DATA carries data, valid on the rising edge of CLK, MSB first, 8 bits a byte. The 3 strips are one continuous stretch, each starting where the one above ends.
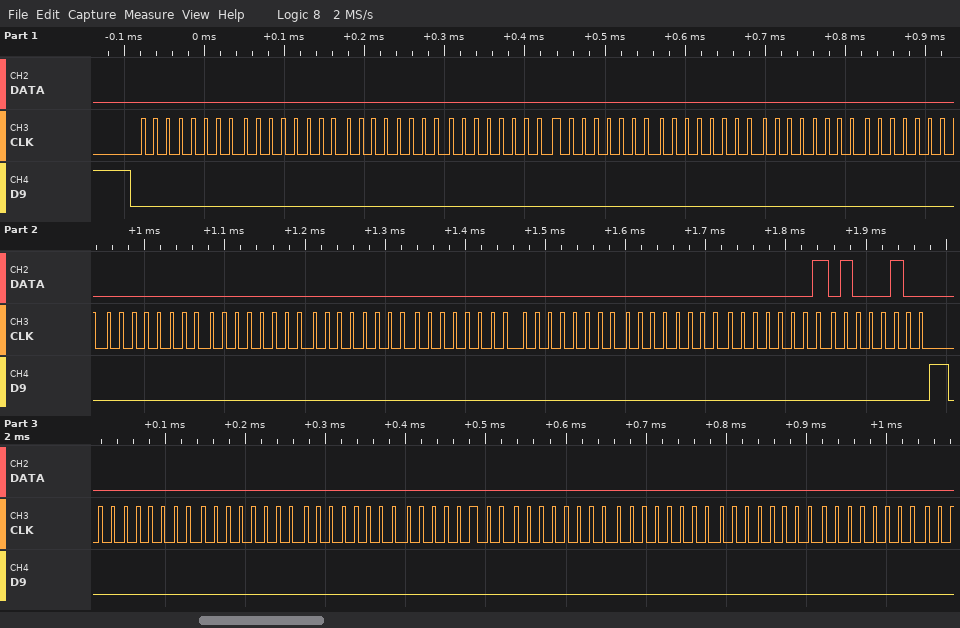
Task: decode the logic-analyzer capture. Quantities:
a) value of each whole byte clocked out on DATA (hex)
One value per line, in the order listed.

00 00 00 00 00 00 00 00 00 00 00 00 00 00 01 44 00 00 00 00 00 00 00 00
